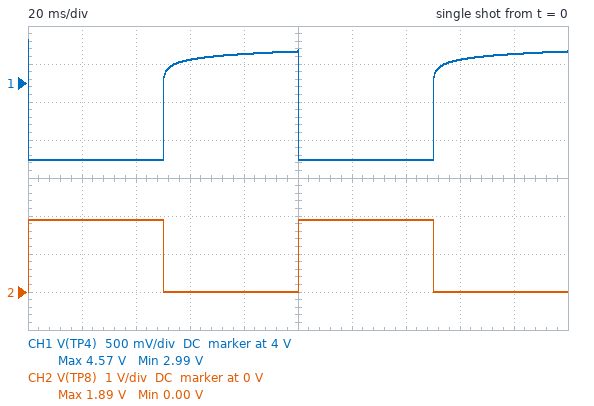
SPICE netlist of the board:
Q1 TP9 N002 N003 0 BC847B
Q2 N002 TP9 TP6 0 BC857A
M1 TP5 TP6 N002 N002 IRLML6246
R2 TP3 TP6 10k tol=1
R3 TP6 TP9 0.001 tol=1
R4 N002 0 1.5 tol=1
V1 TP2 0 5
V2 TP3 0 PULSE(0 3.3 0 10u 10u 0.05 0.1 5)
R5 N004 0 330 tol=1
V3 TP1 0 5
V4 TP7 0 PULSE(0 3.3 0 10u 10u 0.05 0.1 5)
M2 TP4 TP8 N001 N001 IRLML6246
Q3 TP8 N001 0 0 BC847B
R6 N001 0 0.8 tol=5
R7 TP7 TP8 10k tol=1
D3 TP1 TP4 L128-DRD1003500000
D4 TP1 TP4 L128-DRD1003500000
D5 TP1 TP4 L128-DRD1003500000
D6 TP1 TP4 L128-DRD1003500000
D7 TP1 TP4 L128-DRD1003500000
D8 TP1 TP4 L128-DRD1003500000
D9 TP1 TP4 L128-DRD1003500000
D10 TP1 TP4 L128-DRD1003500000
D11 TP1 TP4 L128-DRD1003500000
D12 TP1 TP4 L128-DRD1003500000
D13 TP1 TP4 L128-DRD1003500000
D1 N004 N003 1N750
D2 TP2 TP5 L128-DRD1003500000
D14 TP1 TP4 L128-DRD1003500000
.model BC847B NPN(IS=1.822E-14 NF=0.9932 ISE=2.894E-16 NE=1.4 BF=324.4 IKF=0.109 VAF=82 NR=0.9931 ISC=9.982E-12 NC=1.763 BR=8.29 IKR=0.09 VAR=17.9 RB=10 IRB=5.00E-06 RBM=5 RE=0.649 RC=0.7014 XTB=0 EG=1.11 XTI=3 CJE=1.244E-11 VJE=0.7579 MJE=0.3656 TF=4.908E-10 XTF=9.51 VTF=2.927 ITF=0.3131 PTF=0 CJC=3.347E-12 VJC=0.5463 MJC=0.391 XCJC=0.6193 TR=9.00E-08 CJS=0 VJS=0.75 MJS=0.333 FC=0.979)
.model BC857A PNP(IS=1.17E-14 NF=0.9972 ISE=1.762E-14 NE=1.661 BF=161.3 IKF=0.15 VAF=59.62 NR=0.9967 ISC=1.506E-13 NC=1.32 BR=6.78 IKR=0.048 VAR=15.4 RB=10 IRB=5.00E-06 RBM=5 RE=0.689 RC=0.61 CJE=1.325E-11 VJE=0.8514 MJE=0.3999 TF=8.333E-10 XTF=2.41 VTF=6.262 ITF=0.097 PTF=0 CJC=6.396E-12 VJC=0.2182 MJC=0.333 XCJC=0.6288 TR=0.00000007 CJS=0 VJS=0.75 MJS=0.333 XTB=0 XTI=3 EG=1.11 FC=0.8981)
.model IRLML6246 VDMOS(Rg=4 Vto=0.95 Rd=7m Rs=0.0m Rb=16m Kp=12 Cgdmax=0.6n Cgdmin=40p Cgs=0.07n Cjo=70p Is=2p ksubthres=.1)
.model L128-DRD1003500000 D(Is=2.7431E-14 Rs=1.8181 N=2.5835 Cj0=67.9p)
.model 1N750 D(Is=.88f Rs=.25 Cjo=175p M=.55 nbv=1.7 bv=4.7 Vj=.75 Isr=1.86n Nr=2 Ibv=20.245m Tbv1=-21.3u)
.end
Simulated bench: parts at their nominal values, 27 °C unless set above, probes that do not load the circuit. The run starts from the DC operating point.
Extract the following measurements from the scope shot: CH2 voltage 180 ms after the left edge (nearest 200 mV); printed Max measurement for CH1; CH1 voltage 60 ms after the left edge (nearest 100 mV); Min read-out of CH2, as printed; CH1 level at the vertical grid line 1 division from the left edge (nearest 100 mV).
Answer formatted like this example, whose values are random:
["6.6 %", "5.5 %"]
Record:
["0 V", "4.57 V", "4.3 V", "0.00 V", "3.0 V"]
